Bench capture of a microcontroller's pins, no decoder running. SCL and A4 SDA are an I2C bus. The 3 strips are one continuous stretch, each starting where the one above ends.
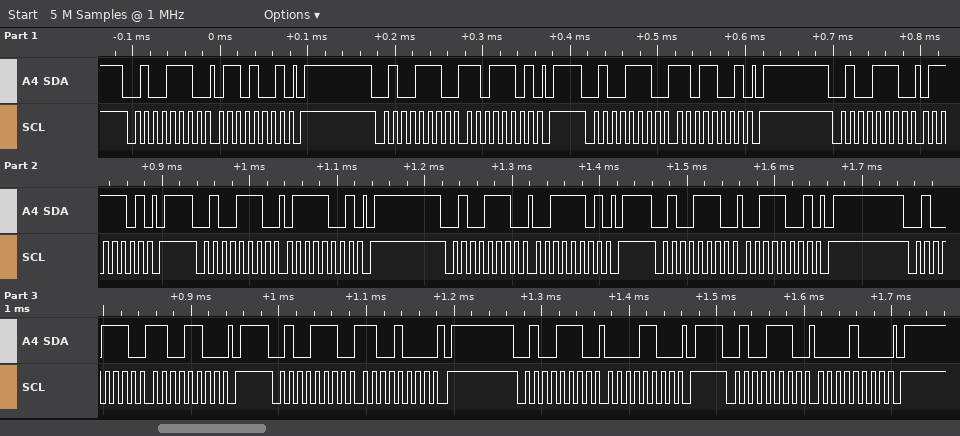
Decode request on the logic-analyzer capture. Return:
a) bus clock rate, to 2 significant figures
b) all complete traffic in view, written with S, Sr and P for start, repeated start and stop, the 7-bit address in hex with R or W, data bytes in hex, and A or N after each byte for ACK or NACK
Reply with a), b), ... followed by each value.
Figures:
a) 100 kHz
b) S 27W A 69 A P S 27W A DD A P S 27W A D9 A P S 27W A 7D A P S 27W A 79 A P S 27W A 3D A P S 27W A 39 A P S 27W A CC A P S 27W A C8 A P S 27W A 0C A P S 27W A 08 A P
